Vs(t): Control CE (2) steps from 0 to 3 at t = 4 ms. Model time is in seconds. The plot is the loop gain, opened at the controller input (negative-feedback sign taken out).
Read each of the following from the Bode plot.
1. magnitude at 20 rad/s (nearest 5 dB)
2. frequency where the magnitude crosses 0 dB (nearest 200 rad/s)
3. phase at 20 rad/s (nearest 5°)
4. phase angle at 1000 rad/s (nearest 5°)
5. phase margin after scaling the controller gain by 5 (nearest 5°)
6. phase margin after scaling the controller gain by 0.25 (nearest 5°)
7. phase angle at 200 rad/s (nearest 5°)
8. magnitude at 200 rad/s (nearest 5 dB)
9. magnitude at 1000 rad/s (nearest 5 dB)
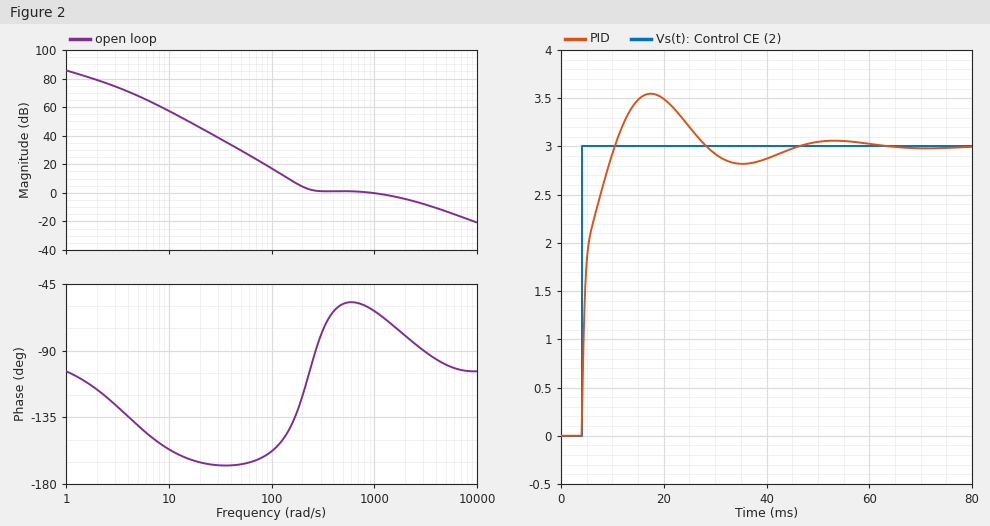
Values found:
45 dB
1000 rad/s
-165°
-65°
80°
30°
-120°
5 dB
0 dB
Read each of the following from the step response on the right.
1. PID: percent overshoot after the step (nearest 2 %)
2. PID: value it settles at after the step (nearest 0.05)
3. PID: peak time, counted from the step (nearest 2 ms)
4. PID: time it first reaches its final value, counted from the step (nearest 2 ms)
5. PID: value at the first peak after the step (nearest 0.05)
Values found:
18 %
3.00
14 ms
6 ms
3.55
